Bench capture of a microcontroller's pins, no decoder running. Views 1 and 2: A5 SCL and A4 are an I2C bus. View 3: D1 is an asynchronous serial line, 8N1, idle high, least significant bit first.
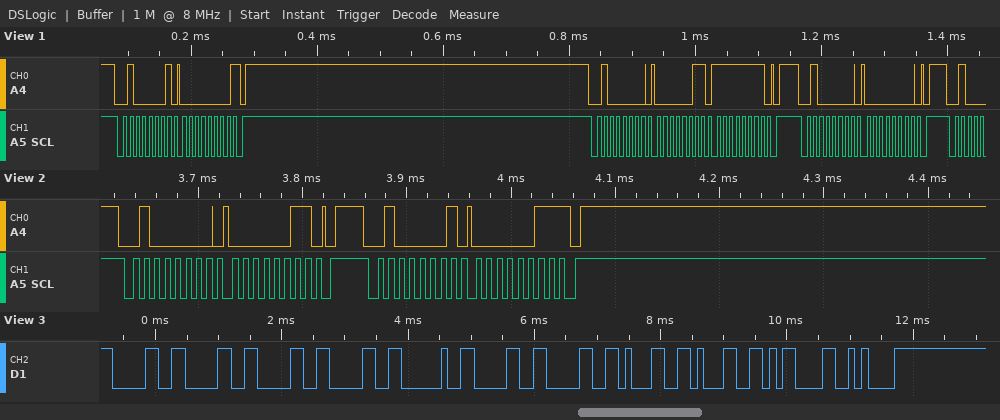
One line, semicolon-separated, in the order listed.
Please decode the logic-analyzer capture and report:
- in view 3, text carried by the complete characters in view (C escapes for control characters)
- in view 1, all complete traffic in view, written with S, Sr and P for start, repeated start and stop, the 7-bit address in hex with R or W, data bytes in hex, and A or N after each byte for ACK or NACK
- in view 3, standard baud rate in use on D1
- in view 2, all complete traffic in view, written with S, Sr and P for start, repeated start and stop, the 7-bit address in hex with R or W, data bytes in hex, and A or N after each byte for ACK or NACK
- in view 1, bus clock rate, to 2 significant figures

"0000 0011\r\n"; S 20R A 00 N P S 20W A 03 A FF A P S 20W A 00 A P; 9600 baud; S 20W A 03 A P S 20R A 03 N P; 100 kHz
